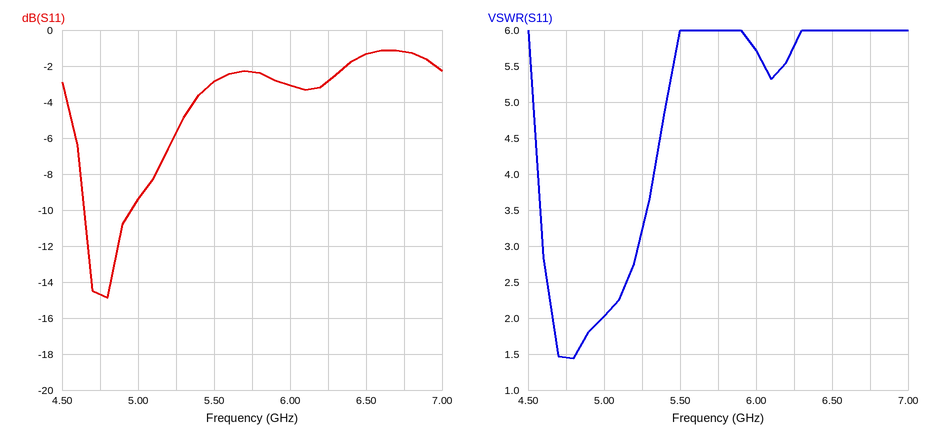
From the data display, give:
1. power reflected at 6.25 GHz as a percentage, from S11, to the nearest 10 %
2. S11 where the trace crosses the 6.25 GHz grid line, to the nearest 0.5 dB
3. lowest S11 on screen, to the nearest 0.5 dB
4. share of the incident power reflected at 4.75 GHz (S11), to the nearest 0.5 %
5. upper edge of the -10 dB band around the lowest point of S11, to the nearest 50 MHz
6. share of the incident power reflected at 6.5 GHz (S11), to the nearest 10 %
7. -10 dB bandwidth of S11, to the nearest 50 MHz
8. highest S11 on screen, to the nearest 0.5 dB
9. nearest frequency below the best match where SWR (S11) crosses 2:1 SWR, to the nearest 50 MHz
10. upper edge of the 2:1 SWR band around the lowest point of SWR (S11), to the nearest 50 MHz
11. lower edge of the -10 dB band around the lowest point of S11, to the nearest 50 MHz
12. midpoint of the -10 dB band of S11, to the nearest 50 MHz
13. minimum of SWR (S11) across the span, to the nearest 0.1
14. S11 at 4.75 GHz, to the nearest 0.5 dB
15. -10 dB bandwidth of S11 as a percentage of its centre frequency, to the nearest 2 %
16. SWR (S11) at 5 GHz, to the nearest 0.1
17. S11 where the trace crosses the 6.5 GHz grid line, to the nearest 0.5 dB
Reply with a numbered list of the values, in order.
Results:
1. 50 %
2. -3.0 dB
3. -15.0 dB
4. 3.5 %
5. 4.95 GHz
6. 70 %
7. 300 MHz
8. -1.0 dB
9. 4.65 GHz
10. 5.00 GHz
11. 4.65 GHz
12. 4.80 GHz
13. 1.4
14. -14.5 dB
15. 6 %
16. 2.0
17. -1.5 dB
